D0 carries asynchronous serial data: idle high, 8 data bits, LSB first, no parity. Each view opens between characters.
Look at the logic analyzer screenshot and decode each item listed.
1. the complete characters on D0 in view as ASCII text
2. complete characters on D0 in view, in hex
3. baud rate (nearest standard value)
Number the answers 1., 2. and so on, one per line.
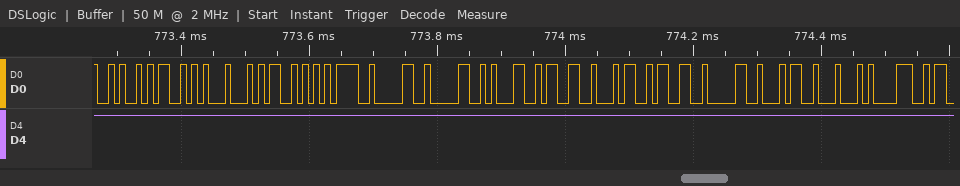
1. "JSDS=00134304D8"
2. 4A, 53, 44, 53, 3D, 30, 30, 31, 33, 34, 33, 30, 34, 44, 38
3. 115200 baud
